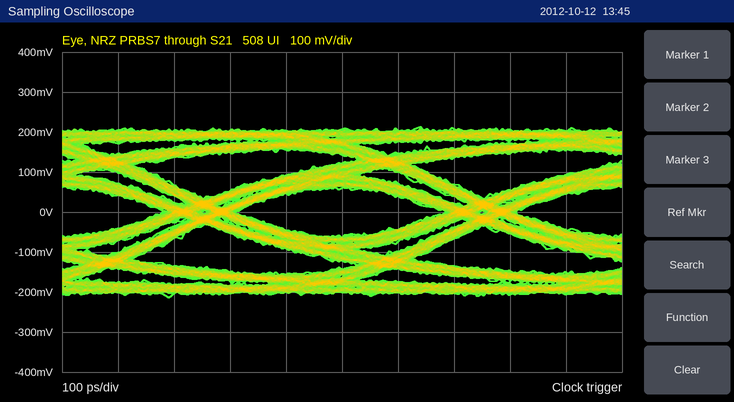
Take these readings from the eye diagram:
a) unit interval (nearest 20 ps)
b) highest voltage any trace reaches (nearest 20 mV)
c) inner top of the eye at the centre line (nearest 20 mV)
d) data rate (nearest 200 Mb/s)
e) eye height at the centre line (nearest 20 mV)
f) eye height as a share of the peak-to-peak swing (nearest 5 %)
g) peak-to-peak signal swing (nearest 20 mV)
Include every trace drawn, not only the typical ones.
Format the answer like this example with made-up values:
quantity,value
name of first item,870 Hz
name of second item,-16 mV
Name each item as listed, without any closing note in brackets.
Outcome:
quantity,value
unit interval,500 ps
highest voltage any trace reaches,220 mV
inner top of the eye at the centre line,60 mV
data rate,2.0 Gb/s
eye height at the centre line,120 mV
eye height as a share of the peak-to-peak swing,30 %
peak-to-peak signal swing,420 mV
